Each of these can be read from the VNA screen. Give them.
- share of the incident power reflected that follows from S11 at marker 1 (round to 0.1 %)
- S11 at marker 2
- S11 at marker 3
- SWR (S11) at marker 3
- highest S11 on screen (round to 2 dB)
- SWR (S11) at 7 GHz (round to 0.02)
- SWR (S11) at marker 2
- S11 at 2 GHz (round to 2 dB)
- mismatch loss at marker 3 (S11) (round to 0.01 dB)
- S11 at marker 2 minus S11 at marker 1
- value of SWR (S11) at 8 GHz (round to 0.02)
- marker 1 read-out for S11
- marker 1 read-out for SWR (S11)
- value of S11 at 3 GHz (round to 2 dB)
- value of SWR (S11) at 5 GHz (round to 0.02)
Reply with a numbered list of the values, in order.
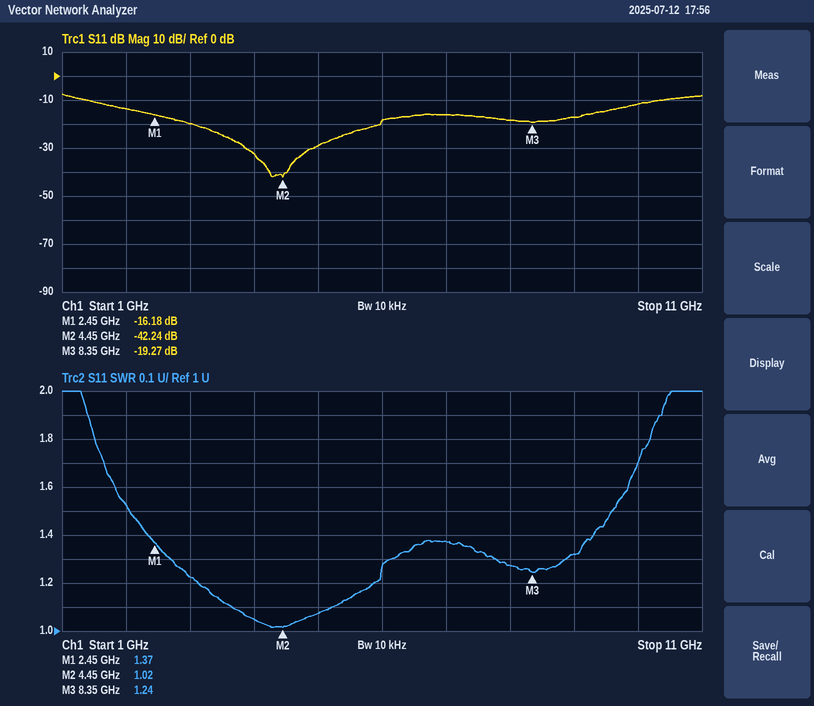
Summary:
1. 2.4 %
2. -42.24 dB
3. -19.27 dB
4. 1.24
5. -8 dB
6. 1.38
7. 1.02
8. -14 dB
9. 0.05 dB
10. -26.06 dB
11. 1.28
12. -16.18 dB
13. 1.37
14. -20 dB
15. 1.08
